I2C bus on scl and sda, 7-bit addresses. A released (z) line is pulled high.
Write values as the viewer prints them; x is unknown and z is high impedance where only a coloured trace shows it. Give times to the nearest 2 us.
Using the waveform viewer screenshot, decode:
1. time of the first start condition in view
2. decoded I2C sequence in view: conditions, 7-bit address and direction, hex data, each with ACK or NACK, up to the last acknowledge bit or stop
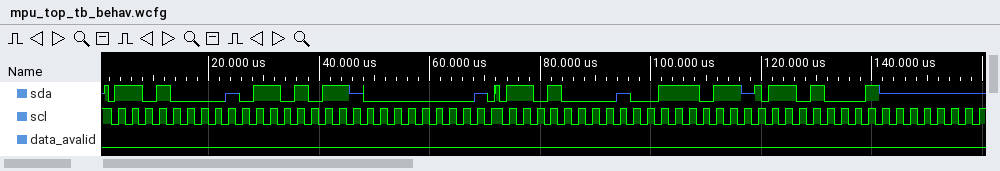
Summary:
2 us
start, address 68 write NACK, 6B NACK, 00 NACK, stop, start, address 68 write NACK, 3B NACK, repeated start, address 68 read NACK
